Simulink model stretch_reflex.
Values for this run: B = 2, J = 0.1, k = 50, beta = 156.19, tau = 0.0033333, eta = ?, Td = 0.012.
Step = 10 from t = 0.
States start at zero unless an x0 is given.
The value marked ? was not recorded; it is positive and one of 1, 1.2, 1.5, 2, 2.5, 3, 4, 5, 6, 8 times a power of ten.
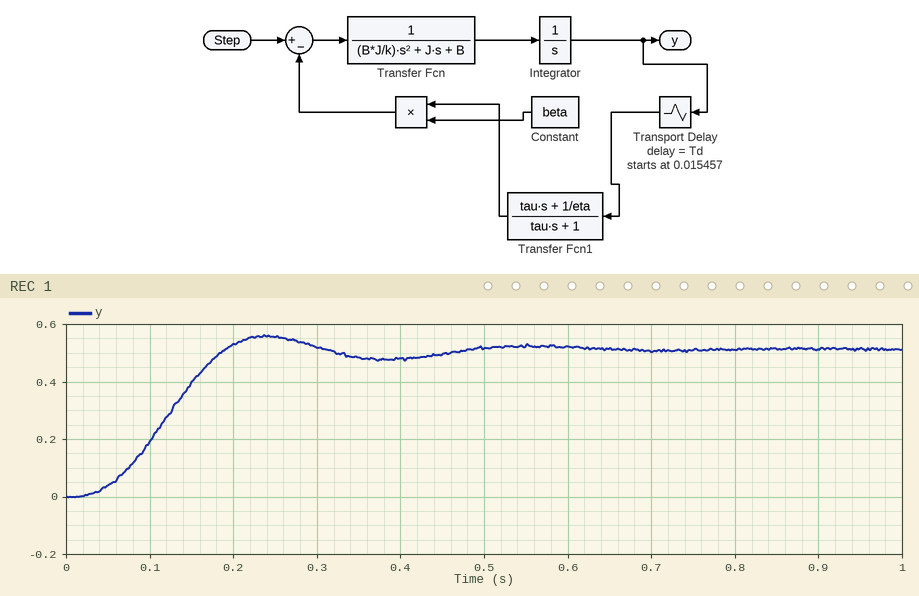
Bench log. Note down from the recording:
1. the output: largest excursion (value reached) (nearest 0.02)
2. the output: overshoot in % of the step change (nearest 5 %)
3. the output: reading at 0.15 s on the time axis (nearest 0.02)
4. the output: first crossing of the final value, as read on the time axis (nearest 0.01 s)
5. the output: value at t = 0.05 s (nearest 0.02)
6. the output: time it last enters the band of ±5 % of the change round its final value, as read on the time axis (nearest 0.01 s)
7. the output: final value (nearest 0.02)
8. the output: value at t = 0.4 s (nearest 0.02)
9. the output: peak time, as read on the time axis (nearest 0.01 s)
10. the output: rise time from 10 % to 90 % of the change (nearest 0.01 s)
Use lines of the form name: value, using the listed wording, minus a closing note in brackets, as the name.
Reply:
the output: largest excursion (value reached): 0.56
the output: overshoot in % of the step change: 10 %
the output: reading at 0.15 s on the time axis: 0.40
the output: first crossing of the final value, as read on the time axis: 0.19 s
the output: value at t = 0.05 s: 0.04
the output: time it last enters the band of ±5 % of the change round its final value, as read on the time axis: 0.43 s
the output: final value: 0.52
the output: value at t = 0.4 s: 0.48
the output: peak time, as read on the time axis: 0.24 s
the output: rise time from 10 % to 90 % of the change: 0.11 s
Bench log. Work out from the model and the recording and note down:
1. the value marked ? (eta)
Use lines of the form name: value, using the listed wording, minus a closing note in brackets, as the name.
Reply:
the value marked ?: 8
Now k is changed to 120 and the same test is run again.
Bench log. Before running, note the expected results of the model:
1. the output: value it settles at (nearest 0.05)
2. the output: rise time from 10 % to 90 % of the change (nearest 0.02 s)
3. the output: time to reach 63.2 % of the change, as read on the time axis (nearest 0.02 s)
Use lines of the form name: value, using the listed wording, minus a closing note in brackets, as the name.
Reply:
the output: value it settles at: 0.50
the output: rise time from 10 % to 90 % of the change: 0.14 s
the output: time to reach 63.2 % of the change, as read on the time axis: 0.12 s
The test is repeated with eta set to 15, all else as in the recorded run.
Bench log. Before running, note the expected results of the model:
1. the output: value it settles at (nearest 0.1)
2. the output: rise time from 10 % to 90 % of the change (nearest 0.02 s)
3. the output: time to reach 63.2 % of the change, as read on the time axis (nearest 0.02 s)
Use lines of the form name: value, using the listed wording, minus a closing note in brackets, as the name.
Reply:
the output: value it settles at: 1.0
the output: rise time from 10 % to 90 % of the change: 0.40 s
the output: time to reach 63.2 % of the change, as read on the time axis: 0.20 s
